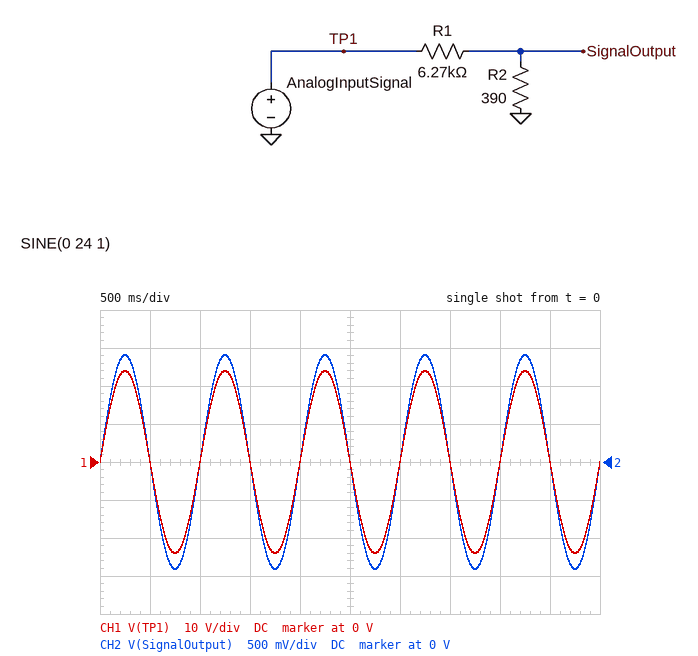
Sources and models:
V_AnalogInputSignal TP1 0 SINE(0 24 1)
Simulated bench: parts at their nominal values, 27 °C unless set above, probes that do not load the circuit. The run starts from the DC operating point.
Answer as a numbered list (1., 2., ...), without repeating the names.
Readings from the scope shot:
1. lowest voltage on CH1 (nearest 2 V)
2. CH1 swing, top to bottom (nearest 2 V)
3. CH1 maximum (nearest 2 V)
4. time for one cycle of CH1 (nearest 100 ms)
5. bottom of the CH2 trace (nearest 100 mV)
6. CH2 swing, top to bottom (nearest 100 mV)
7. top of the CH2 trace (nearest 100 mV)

1. -24 V
2. 48 V
3. 24 V
4. 1.0 s
5. -1.4 V
6. 2.8 V
7. 1.4 V
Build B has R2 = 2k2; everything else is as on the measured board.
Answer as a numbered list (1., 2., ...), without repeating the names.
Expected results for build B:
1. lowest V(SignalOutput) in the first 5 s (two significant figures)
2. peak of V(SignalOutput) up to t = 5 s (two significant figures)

1. -6.2 V
2. 6.2 V
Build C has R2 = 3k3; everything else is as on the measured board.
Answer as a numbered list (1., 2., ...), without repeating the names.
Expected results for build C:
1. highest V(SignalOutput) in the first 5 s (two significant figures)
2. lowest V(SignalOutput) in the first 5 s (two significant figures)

1. 8.3 V
2. -8.3 V
